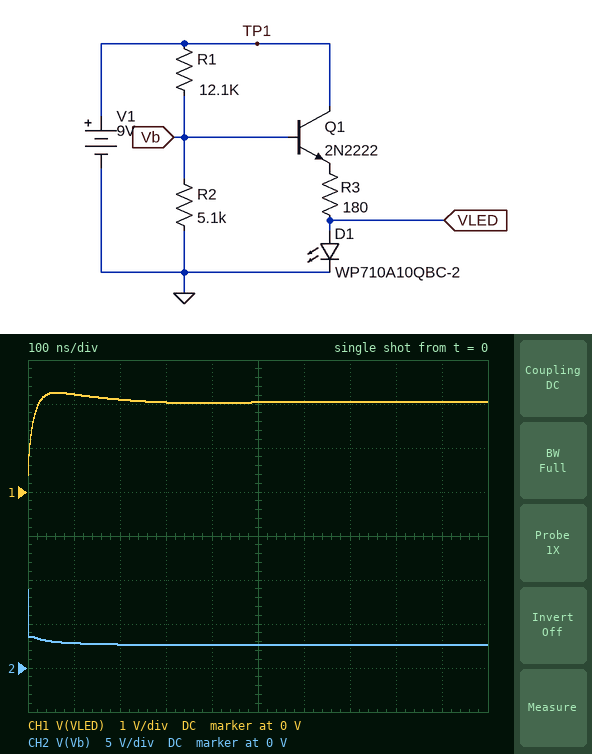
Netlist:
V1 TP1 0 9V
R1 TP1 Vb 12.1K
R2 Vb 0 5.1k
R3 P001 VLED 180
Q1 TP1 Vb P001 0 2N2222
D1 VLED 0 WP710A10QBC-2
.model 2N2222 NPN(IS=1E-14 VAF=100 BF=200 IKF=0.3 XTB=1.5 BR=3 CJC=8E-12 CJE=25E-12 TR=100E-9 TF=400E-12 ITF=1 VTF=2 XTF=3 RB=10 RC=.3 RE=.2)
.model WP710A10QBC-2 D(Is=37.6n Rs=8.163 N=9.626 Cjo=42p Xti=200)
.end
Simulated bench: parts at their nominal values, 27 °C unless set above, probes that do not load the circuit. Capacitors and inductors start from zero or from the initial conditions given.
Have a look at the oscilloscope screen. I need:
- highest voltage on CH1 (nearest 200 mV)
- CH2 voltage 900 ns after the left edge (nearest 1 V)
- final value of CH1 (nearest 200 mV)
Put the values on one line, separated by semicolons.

2.2 V; 3 V; 2.0 V
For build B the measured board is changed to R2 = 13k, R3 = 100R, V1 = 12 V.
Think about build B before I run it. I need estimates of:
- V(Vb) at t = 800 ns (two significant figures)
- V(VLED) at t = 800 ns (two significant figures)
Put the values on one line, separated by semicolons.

5.7 V; 3.4 V
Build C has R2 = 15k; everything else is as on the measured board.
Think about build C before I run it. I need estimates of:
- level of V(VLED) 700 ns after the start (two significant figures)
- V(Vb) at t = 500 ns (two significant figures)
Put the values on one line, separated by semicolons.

3.0 V; 4.8 V
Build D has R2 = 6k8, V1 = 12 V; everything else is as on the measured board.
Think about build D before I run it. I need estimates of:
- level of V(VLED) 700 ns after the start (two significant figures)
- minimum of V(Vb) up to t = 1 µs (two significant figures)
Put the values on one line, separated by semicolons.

2.9 V; 4.2 V
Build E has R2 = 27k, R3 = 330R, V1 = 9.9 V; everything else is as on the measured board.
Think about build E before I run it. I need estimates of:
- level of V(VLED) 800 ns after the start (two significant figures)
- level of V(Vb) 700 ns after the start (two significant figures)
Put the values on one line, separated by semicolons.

3.1 V; 6.5 V
